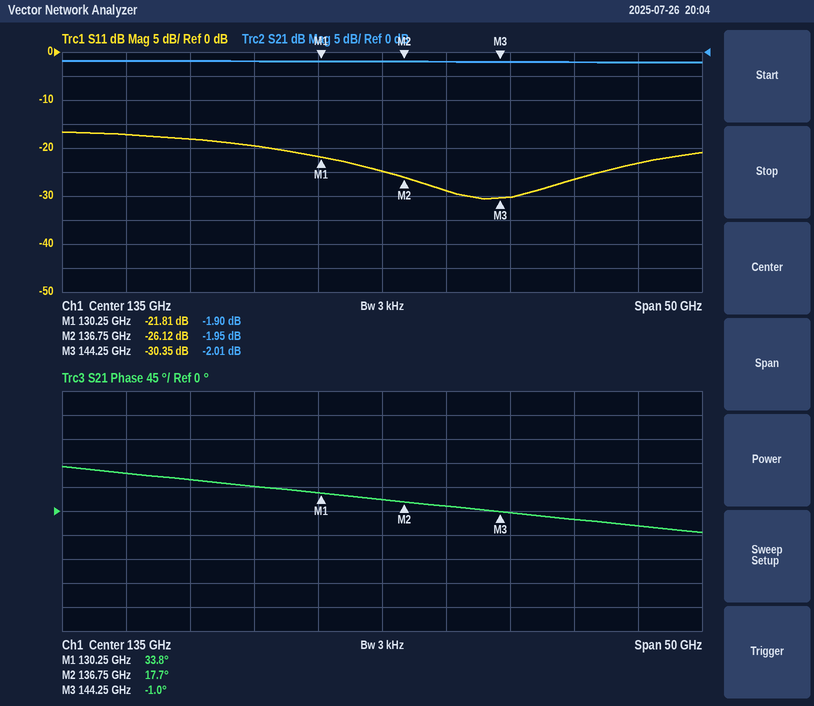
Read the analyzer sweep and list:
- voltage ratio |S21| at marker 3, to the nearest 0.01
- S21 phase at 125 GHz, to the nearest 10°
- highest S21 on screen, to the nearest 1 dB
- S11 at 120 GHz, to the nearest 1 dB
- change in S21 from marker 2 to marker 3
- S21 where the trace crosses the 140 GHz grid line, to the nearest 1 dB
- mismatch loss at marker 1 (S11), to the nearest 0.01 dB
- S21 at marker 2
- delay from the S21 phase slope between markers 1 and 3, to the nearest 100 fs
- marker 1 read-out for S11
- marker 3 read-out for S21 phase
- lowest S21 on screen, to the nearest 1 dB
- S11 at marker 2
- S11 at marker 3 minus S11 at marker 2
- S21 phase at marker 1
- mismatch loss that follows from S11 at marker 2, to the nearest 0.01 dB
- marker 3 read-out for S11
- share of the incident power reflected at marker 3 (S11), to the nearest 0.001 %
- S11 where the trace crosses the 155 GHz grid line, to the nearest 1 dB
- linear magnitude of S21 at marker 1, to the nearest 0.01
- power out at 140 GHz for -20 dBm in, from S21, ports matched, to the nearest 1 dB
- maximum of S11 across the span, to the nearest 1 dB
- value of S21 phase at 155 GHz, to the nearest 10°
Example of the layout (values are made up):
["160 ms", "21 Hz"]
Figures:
["0.79", "50°", "-2 dB", "-18 dB", "-0.06 dB", "-2 dB", "0.03 dB", "-1.95 dB", "6.9 ps", "-21.81 dB", "-1.0°", "-2 dB", "-26.12 dB", "-4.23 dB", "33.8°", "0.01 dB", "-30.35 dB", "0.092 %", "-23 dB", "0.80", "-22 dBm", "-17 dB", "-30°"]
